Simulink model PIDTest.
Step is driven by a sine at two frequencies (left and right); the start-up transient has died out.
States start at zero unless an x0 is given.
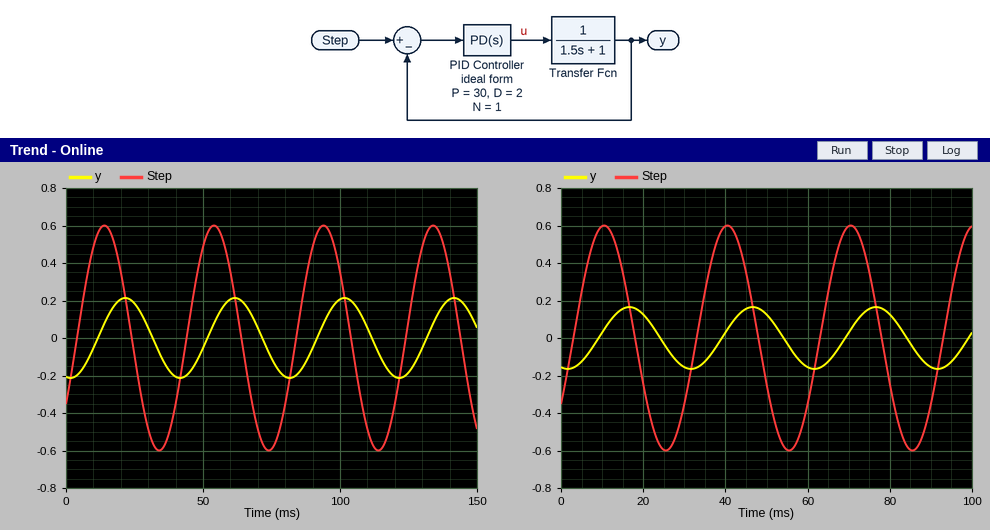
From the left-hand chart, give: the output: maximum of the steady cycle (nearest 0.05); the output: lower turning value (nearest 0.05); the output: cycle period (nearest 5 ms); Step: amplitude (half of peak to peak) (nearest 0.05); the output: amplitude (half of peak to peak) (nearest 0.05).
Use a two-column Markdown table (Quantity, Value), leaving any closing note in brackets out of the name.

| Quantity | Value |
|---|---|
| the output: maximum of the steady cycle | 0.20 |
| the output: lower turning value | -0.20 |
| the output: cycle period | 40 ms |
| Step: amplitude (half of peak to peak) | 0.60 |
| the output: amplitude (half of peak to peak) | 0.20 |
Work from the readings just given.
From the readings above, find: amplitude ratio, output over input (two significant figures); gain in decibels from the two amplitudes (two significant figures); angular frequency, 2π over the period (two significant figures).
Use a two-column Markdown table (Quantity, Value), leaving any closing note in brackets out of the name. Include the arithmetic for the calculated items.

| Quantity | Value |
|---|---|
| amplitude ratio, output over input | 0.2 / 0.6 = 0.33 |
| gain in decibels from the two amplitudes | 20 log10(0.2 / 0.6) = -9.5 dB |
| angular frequency, 2π over the period | 2π / 40 = 0.16 rad/ms |
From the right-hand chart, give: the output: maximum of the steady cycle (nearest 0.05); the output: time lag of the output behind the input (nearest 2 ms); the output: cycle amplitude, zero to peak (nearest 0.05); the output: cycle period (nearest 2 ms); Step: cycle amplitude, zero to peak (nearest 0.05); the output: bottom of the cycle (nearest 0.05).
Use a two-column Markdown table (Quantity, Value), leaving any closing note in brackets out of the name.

| Quantity | Value |
|---|---|
| the output: maximum of the steady cycle | 0.15 |
| the output: time lag of the output behind the input | 6 ms |
| the output: cycle amplitude, zero to peak | 0.15 |
| the output: cycle period | 30 ms |
| Step: cycle amplitude, zero to peak | 0.60 |
| the output: bottom of the cycle | -0.15 |
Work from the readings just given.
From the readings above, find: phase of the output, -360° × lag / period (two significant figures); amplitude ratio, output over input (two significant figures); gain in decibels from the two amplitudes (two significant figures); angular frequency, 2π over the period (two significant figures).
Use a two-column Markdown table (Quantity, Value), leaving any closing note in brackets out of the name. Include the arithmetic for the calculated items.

| Quantity | Value |
|---|---|
| phase of the output, -360° × lag / period | -360 × 6 / 30 = -72° |
| amplitude ratio, output over input | 0.15 / 0.6 = 0.25 |
| gain in decibels from the two amplitudes | 20 log10(0.15 / 0.6) = -12 dB |
| angular frequency, 2π over the period | 2π / 30 = 0.21 rad/ms |
